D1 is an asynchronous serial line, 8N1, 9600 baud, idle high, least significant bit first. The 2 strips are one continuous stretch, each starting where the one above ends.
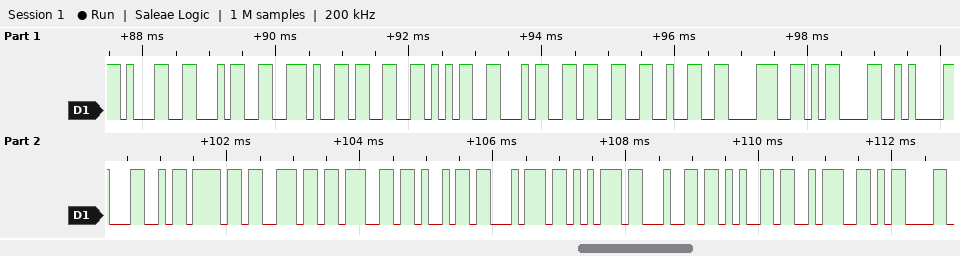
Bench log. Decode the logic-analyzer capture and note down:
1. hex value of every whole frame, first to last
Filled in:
31 34 2E 33 35 34 33 32 38 0D 0A 4C 6F 6E 67 69 74 75 64 65 3A 0D
